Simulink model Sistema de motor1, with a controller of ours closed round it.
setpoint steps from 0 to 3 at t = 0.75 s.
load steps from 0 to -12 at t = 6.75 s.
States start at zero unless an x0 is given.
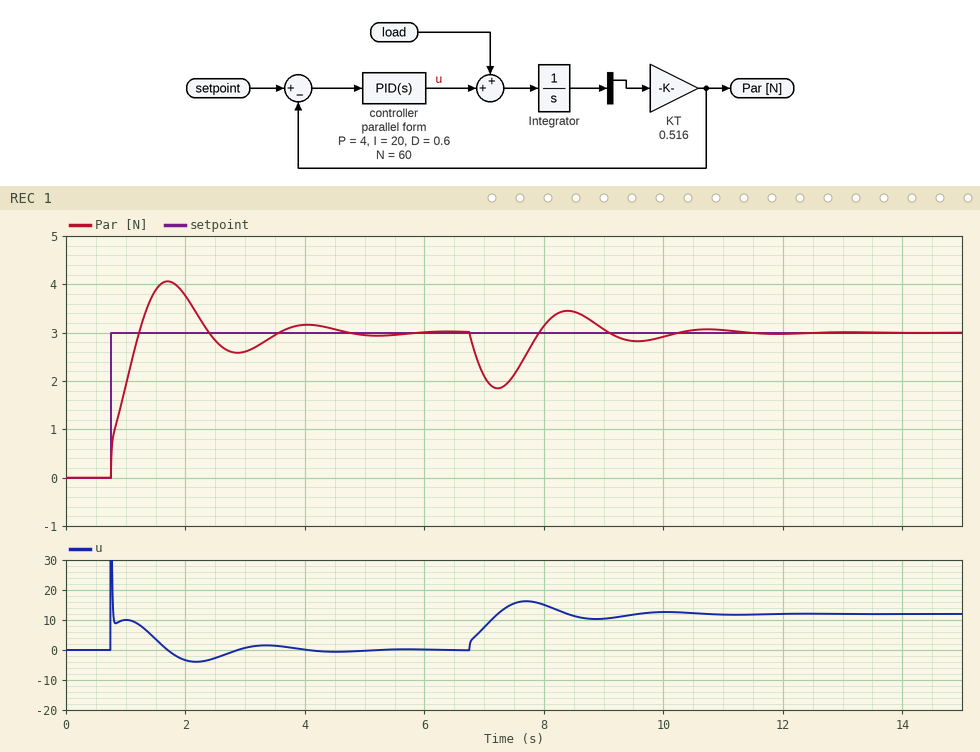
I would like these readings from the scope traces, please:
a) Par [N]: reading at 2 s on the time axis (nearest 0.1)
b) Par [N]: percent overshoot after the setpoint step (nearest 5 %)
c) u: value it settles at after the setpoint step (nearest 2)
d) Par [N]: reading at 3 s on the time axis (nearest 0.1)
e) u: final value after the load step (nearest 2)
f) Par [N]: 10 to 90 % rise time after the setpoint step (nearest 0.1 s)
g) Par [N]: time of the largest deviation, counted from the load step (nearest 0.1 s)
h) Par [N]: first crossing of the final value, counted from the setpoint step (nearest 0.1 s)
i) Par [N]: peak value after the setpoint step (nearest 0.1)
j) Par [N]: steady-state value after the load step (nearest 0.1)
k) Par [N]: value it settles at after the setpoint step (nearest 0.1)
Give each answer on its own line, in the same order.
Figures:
3.8
35 %
0
2.6
12
0.4 s
0.5 s
0.5 s
4.1
3.0
3.0
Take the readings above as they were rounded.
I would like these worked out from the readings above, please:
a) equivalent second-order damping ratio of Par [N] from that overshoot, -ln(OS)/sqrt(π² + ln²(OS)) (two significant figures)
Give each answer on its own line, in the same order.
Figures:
0.32
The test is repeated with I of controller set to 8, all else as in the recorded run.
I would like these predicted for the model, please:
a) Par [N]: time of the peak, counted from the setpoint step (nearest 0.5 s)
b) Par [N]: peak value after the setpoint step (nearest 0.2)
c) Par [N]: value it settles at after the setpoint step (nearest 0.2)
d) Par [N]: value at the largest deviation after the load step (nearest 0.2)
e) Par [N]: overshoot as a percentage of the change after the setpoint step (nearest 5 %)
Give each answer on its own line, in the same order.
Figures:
1.5 s
3.8
3.0
1.4
25 %
